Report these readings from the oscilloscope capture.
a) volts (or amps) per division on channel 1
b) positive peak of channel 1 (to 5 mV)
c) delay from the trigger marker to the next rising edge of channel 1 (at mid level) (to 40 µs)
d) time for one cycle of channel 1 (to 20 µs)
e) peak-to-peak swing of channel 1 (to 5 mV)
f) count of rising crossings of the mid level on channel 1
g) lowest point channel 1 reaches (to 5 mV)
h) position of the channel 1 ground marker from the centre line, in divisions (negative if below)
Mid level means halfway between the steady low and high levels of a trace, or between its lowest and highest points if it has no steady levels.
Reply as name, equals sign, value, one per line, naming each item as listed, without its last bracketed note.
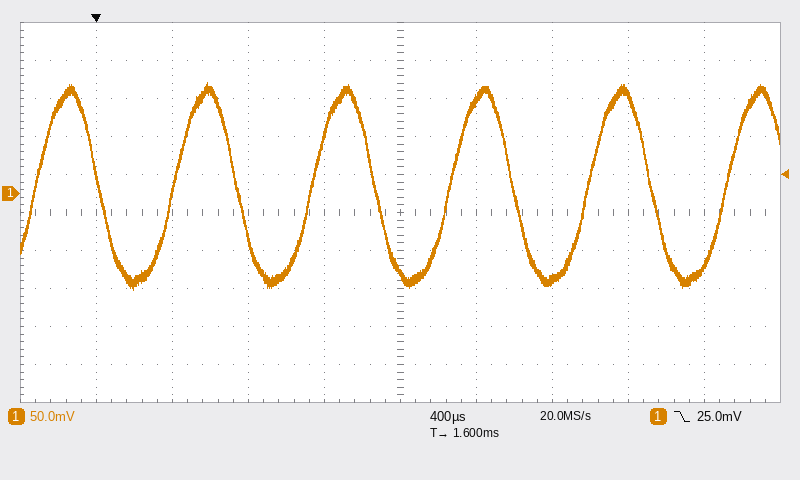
volts (or amps) per division on channel 1 = 50 mV
positive peak of channel 1 = 145 mV
delay from the trigger marker to the next rising edge of channel 1 (at mid level) = 400 µs
time for one cycle of channel 1 = 720 µs
peak-to-peak swing of channel 1 = 270 mV
count of rising crossings of the mid level on channel 1 = 6
lowest point channel 1 reaches = -125 mV
position of the channel 1 ground marker from the centre line, in divisions = +0.5 div
